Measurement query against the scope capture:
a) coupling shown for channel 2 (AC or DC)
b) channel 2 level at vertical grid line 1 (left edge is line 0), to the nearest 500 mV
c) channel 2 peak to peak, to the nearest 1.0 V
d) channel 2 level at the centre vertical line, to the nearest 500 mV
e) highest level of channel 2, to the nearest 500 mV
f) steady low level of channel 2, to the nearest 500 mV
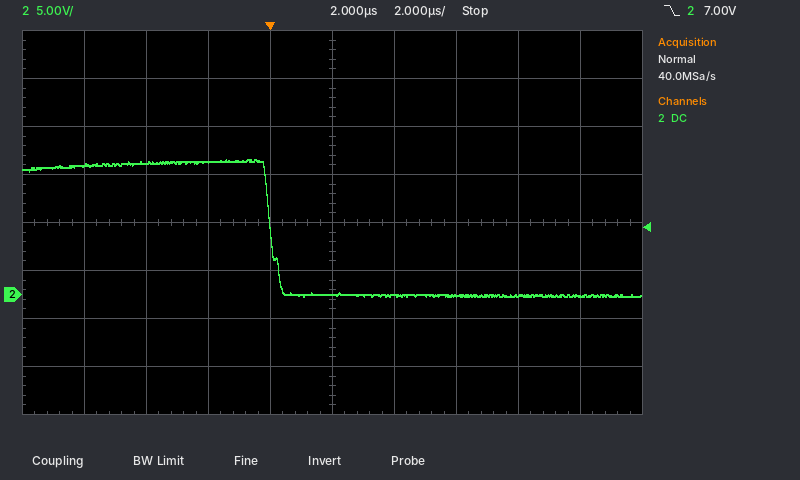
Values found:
DC
13.5 V
14.0 V
0.0 V
14.0 V
0.0 V
